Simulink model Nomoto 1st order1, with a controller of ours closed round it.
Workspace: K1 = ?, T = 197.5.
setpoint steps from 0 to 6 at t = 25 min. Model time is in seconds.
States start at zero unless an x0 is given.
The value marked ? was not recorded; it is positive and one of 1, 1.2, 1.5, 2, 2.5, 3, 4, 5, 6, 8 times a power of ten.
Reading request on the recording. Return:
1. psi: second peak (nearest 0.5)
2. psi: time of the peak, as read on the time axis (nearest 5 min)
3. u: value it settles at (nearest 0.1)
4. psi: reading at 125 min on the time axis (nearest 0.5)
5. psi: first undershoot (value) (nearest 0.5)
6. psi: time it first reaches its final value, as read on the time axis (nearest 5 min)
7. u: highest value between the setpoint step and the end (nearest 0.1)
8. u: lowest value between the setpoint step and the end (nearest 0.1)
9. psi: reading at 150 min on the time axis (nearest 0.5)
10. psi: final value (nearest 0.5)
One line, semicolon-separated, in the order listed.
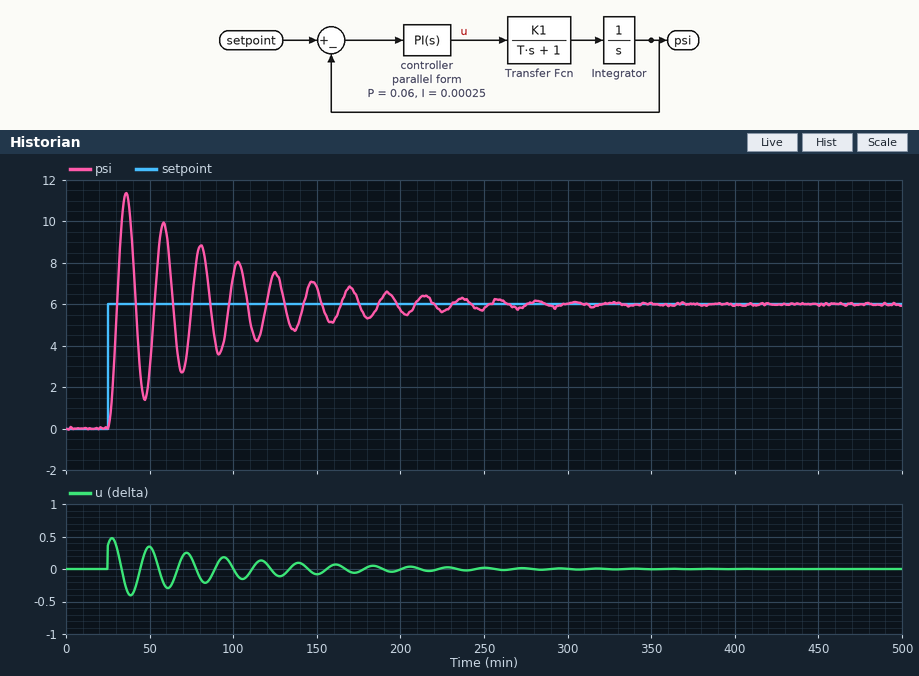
10.0; 35 min; 0.0; 7.5; 1.5; 30 min; 0.5; -0.4; 7.0; 6.0
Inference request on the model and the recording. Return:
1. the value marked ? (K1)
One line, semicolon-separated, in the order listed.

0.08
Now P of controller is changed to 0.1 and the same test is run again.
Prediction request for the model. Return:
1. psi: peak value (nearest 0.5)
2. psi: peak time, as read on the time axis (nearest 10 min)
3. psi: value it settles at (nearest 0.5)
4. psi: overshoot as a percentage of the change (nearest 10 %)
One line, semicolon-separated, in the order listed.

10.0; 30 min; 6.0; 70 %
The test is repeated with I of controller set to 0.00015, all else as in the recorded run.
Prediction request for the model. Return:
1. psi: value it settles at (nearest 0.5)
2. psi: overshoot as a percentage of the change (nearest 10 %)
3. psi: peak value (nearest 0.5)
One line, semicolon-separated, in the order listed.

6.0; 70 %; 10.0
